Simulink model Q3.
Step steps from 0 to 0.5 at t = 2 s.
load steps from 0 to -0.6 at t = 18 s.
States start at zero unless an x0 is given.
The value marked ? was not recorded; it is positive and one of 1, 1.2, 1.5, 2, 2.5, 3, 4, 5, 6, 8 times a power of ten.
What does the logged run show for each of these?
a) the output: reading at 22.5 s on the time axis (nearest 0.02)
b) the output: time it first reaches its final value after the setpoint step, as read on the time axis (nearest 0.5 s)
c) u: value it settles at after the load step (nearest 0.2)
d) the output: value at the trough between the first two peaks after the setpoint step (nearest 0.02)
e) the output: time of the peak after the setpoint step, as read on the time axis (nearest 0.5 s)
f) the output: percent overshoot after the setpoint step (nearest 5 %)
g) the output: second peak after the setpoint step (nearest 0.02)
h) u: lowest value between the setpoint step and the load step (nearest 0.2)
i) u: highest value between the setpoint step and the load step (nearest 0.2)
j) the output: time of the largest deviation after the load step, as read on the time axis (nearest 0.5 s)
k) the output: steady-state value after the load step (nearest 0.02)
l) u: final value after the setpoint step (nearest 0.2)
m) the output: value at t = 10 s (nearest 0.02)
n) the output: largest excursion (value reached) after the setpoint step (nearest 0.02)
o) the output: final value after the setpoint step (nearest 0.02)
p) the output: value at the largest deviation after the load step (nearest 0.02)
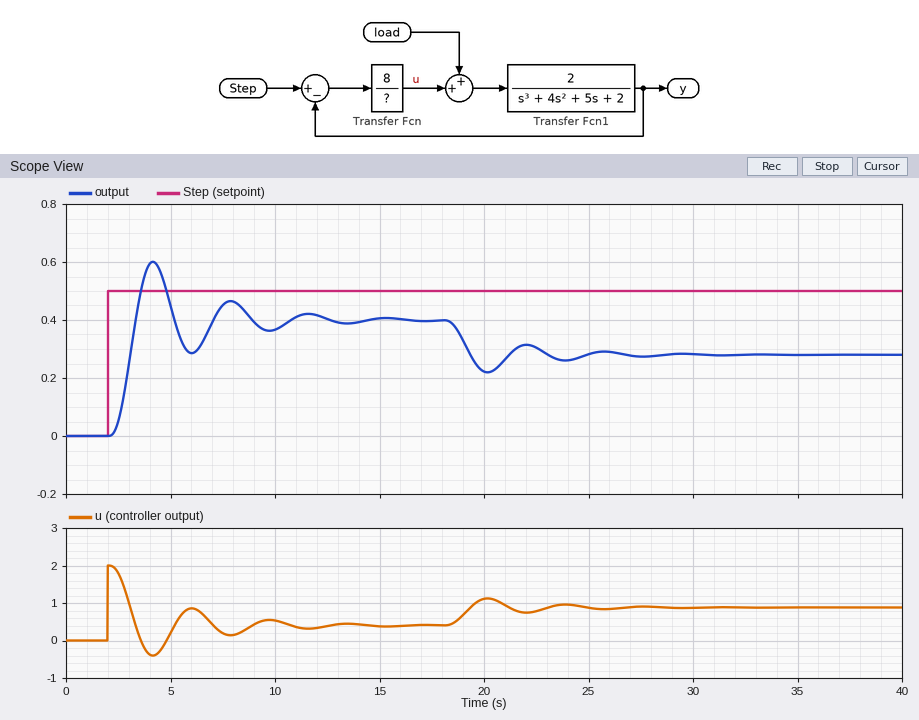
0.30
3.5 s
0.8
0.28
4.0 s
50 %
0.46
-0.4
2.0
20.0 s
0.28
0.4
0.36
0.60
0.40
0.22
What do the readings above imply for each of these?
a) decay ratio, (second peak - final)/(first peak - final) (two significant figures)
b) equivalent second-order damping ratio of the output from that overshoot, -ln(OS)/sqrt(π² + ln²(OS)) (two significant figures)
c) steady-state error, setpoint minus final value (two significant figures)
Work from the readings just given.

0.30
0.22
0.10
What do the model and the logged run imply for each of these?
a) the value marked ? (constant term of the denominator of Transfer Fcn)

2
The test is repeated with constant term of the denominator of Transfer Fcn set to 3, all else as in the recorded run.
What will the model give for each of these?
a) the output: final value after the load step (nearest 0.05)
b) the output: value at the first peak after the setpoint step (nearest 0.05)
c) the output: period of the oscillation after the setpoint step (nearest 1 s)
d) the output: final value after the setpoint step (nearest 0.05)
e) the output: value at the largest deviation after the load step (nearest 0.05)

0.20
0.50
4 s
0.35
0.15
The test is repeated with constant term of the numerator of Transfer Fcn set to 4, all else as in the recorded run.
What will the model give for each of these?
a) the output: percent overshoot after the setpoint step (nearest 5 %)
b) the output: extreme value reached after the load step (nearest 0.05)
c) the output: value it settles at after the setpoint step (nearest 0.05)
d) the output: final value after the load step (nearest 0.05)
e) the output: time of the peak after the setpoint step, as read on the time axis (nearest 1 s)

25 %
0.10
0.35
0.15
5 s
